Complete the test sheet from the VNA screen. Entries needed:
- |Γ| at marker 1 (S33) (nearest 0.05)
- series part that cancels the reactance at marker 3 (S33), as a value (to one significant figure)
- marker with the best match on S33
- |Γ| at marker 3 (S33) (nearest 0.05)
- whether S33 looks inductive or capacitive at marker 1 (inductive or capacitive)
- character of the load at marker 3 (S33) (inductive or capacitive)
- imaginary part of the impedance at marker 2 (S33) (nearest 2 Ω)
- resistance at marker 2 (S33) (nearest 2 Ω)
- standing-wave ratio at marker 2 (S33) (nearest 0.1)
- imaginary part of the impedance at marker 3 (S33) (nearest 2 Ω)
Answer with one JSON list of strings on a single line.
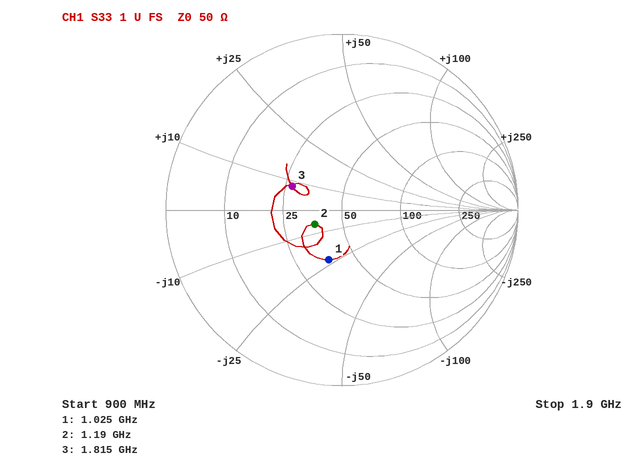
["0.30", "10 pF", "marker 2", "0.30", "capacitive", "inductive", "-6 Ω", "36 Ω", "1.4", "+8 Ω"]
